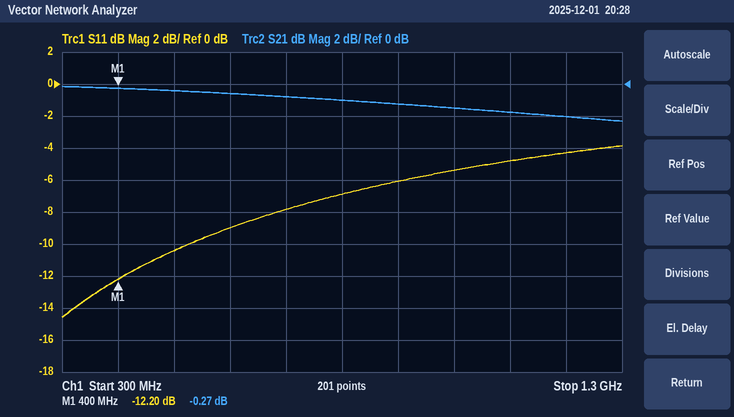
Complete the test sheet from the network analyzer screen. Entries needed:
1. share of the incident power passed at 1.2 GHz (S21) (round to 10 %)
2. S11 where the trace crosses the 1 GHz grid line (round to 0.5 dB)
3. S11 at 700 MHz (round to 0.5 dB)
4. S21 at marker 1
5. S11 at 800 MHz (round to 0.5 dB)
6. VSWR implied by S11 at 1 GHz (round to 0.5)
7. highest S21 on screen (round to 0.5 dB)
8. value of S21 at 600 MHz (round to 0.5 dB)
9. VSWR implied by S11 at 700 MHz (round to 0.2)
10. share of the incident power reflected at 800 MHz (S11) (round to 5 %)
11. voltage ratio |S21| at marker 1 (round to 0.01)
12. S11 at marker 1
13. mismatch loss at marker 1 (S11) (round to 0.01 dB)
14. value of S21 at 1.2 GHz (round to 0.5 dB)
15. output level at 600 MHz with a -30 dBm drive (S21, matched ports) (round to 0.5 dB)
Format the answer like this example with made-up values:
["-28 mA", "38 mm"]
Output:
["60 %", "-5.5 dB", "-8.0 dB", "-0.27 dB", "-7.0 dB", "3.5", "0.0 dB", "-0.5 dB", "2.4", "20 %", "0.97", "-12.20 dB", "0.27 dB", "-2.0 dB", "-30.5 dBm"]
